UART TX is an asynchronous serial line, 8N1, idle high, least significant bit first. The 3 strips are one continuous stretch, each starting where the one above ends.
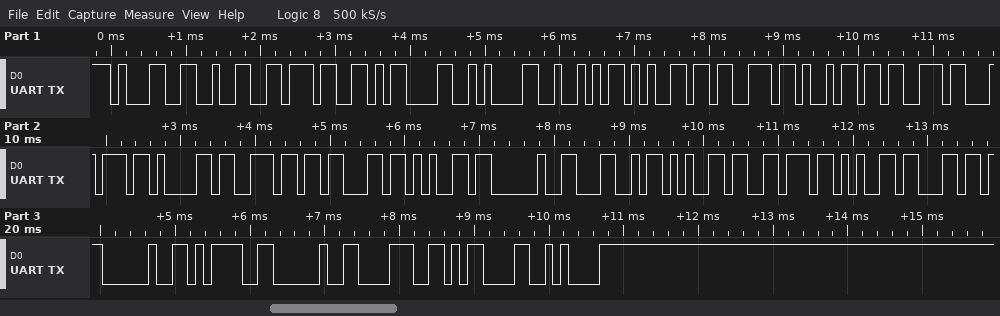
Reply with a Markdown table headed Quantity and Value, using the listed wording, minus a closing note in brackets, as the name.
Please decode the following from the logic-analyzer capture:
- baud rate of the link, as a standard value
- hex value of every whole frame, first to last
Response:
| Quantity | Value |
|---|---|
| baud rate of the link, as a standard value | 9600 baud |
| hex value of every whole frame, first to last | 31 32 37 0D 0A 52 65 73 69 73 74 61 6E 63 65 20 4C 65 76 65 6C 20 3D 20 38 0D 0A |
